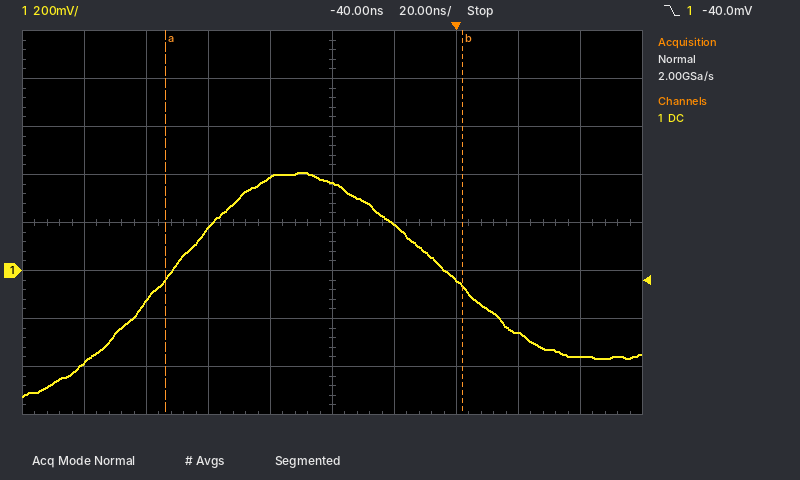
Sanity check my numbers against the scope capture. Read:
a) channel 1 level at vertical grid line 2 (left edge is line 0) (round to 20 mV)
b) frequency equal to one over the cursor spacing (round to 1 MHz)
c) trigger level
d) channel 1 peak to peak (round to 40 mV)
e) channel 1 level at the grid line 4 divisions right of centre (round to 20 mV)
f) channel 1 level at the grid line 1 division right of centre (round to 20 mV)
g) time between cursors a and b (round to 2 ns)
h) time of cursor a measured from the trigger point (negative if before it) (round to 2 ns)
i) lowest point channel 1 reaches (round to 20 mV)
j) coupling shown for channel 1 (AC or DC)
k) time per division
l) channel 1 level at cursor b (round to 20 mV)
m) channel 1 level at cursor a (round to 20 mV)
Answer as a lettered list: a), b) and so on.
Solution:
a) -120 mV
b) 10 MHz
c) -40.0 mV
d) 920 mV
e) -360 mV
f) 200 mV
g) 96 ns
h) -94 ns
i) -520 mV
j) DC
k) 20 ns
l) -60 mV
m) -40 mV
